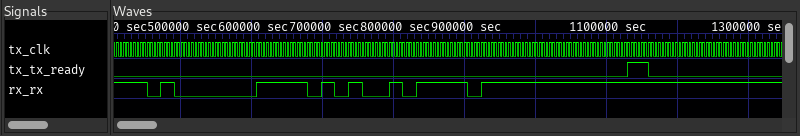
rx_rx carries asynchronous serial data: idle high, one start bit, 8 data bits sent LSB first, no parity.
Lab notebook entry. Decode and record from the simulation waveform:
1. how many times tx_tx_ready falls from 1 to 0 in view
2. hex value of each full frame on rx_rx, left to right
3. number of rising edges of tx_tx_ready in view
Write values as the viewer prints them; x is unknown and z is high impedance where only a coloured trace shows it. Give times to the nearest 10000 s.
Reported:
1
81, A5, FF
1
